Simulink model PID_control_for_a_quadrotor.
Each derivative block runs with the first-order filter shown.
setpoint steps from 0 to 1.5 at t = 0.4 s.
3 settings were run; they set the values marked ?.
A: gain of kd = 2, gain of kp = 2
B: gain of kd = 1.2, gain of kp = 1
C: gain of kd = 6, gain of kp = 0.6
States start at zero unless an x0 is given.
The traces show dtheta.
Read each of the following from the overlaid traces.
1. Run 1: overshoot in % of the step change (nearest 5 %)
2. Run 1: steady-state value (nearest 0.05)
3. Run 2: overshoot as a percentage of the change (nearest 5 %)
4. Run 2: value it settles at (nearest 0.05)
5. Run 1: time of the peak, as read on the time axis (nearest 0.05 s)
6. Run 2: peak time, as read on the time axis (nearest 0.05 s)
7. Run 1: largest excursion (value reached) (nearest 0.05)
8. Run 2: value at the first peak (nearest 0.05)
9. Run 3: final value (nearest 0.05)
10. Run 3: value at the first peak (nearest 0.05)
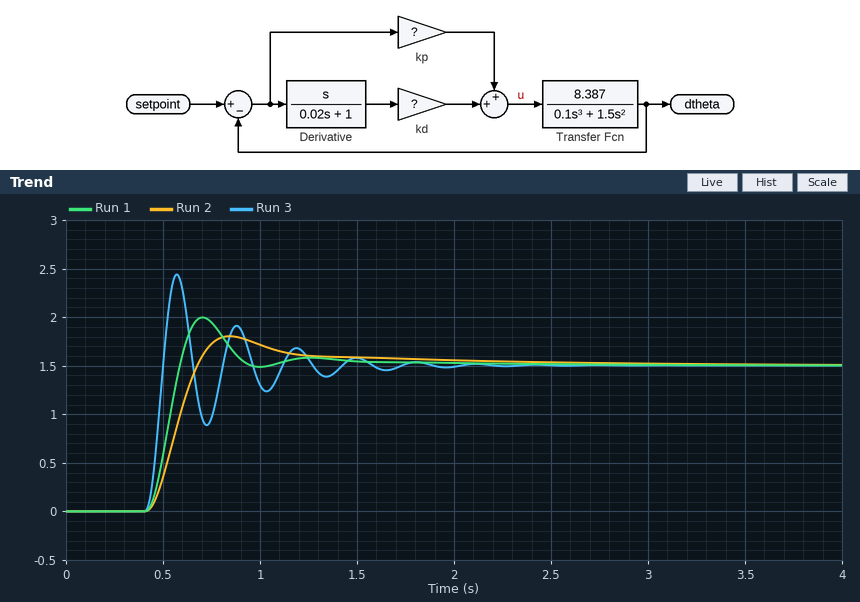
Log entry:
35 %
1.50
20 %
1.50
0.70 s
0.85 s
2.00
1.80
1.50
2.45
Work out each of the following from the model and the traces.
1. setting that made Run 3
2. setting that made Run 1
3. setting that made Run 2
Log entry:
C
A
B
